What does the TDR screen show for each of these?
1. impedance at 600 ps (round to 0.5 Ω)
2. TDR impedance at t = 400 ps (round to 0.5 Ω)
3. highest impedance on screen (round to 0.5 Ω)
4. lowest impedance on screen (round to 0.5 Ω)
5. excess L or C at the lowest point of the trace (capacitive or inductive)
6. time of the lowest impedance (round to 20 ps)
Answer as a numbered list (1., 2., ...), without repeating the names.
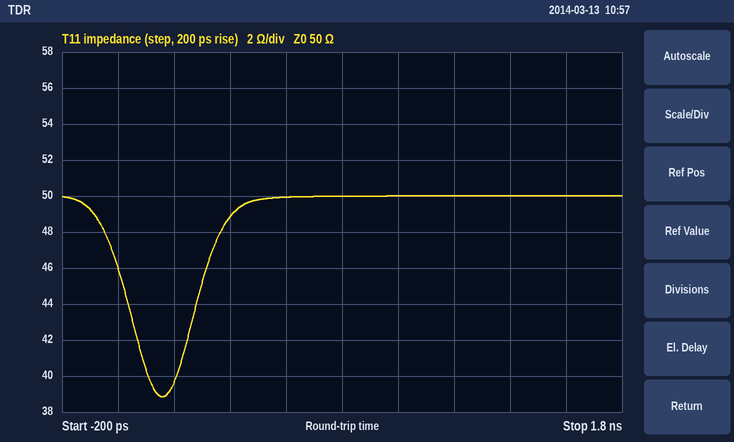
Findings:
1. 50.0 Ω
2. 49.0 Ω
3. 50.0 Ω
4. 39.0 Ω
5. capacitive
6. 160 ps
